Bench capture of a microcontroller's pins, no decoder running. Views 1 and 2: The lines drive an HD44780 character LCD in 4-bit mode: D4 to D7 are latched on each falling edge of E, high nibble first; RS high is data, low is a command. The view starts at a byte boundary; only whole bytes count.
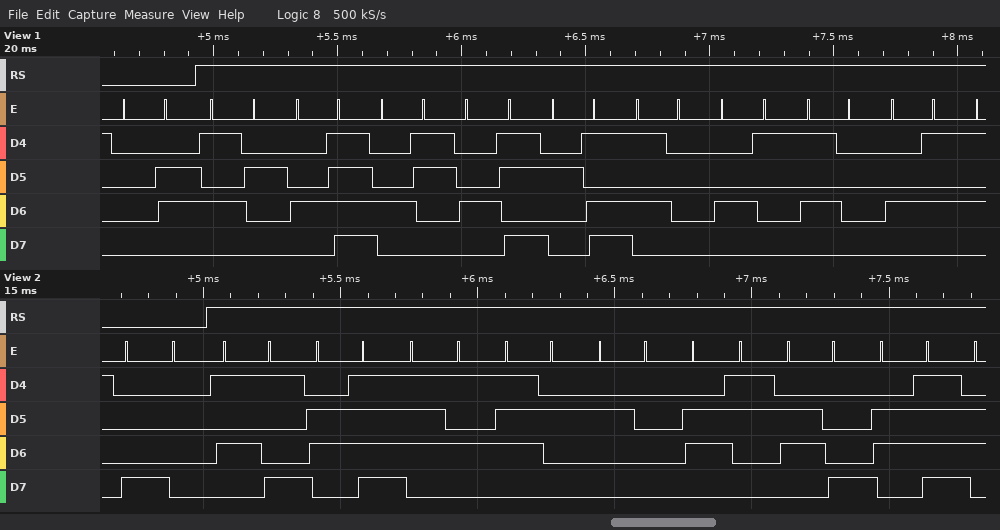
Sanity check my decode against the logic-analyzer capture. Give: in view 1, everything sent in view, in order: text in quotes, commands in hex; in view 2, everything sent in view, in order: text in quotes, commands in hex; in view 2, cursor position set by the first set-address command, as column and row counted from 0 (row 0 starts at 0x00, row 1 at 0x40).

0x06 "ROCK-PAPE"
0x80 "Your cho"
column 0, row 0
